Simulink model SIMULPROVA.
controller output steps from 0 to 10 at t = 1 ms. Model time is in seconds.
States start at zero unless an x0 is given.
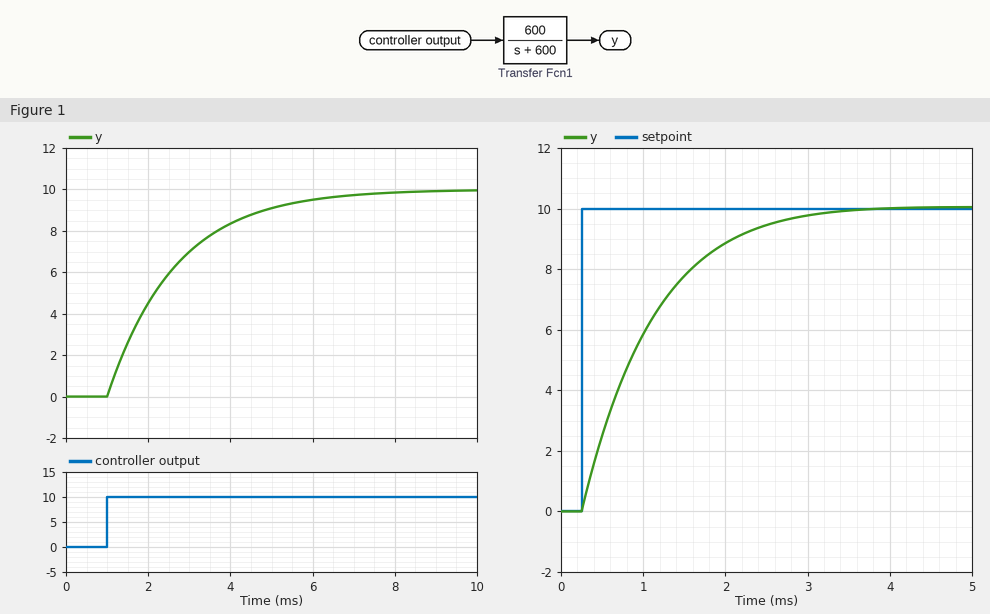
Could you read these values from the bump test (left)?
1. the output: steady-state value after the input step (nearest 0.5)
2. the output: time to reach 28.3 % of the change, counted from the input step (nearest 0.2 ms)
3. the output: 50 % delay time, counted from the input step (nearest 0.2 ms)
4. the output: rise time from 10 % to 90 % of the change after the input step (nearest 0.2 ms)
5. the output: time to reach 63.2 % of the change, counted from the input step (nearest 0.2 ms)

10.0
0.6 ms
1.2 ms
3.6 ms
1.6 ms
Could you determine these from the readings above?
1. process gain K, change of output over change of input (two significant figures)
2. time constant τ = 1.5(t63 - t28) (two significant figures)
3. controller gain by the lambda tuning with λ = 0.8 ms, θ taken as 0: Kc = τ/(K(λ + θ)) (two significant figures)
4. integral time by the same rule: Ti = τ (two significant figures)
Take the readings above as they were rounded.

1.0
1.5 ms
1.9
1.5 ms
